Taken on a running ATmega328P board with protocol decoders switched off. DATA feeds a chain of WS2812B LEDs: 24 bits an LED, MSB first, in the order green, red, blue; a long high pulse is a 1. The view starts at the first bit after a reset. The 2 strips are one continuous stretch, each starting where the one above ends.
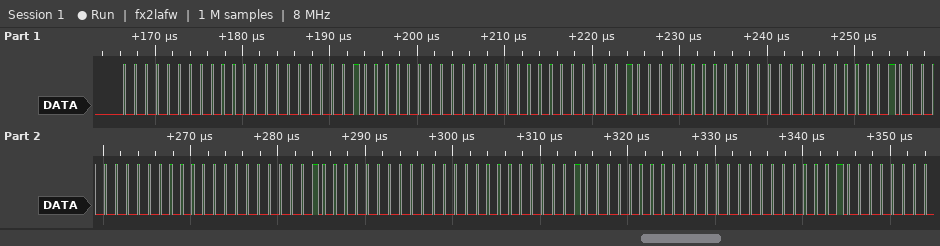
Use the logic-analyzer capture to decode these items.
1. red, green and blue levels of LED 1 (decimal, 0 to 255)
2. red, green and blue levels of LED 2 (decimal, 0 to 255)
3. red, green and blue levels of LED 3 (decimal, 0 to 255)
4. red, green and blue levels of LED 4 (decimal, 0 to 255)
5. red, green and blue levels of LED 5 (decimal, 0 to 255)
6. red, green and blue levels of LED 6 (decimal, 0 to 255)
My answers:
0, 0, 4
0, 0, 2
0, 0, 2
0, 0, 2
0, 0, 2
0, 0, 2
